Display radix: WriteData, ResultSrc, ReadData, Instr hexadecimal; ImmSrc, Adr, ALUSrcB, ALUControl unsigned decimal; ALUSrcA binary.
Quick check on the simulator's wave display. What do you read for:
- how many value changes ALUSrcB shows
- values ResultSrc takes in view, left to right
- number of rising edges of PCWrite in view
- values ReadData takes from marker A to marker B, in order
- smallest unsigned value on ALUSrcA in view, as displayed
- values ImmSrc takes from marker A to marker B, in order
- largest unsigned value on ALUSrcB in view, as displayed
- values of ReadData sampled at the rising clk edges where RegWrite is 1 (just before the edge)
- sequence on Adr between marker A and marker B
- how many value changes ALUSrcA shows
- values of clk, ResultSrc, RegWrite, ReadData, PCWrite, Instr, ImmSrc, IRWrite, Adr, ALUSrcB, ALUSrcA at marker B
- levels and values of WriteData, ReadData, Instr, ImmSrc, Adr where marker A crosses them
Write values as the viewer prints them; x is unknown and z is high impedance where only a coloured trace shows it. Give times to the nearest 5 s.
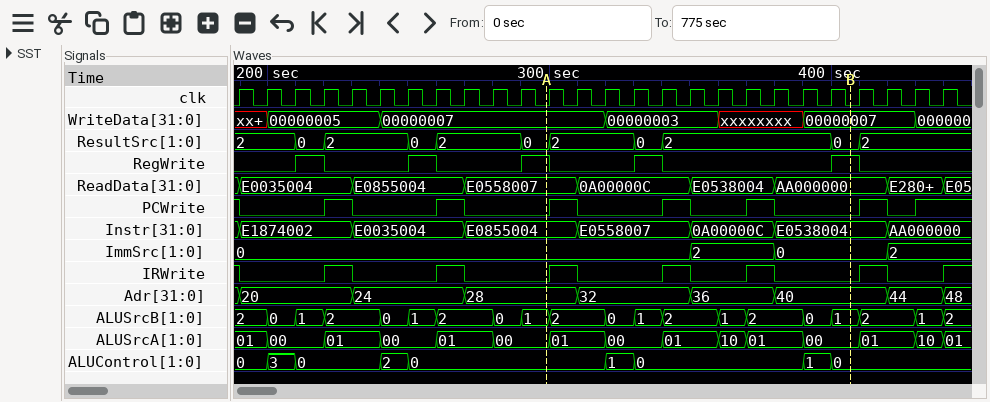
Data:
19
2, 0, 2, 0, 2, 0, 2, 0, 2, 0, 2
7
E0558007, 0A00000C, E0538004, AA000000
00
0, 2, 0
2
E0035004, E0855004, E0558007, 0A00000C, AA000000
28, 32, 36, 40
14
clk=0, ResultSrc=0, RegWrite=1, ReadData=AA000000, PCWrite=0, Instr=E0538004, ImmSrc=0, IRWrite=0, Adr=40, ALUSrcB=1, ALUSrcA=00
WriteData=00000007, ReadData=E0558007, Instr=E0855004, ImmSrc=0, Adr=28
